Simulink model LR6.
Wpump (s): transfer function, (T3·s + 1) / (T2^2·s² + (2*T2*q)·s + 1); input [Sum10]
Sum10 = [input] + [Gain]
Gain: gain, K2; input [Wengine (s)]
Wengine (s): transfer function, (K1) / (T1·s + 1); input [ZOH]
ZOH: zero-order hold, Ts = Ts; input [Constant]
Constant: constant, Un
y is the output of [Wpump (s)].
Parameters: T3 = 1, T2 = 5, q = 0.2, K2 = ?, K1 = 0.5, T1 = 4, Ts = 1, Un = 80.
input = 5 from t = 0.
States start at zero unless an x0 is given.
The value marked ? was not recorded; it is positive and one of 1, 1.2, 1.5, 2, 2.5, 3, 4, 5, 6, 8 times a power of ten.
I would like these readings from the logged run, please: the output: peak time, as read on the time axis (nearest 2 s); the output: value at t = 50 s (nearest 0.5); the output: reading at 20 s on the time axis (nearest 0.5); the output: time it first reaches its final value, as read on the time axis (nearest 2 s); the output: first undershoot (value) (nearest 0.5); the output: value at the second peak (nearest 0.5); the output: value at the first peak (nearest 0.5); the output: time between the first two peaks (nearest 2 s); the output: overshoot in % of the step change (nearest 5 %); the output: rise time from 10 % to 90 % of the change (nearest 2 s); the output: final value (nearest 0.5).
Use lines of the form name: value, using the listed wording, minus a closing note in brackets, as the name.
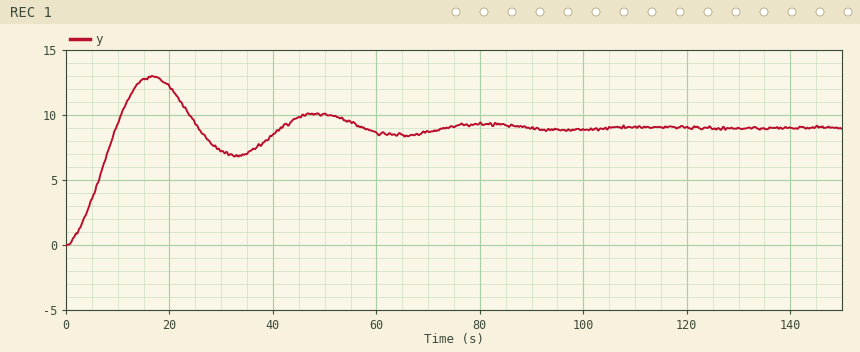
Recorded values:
the output: peak time, as read on the time axis: 16 s
the output: value at t = 50 s: 10.0
the output: reading at 20 s on the time axis: 12.0
the output: time it first reaches its final value, as read on the time axis: 10 s
the output: first undershoot (value): 7.0
the output: value at the second peak: 10.0
the output: value at the first peak: 13.0
the output: time between the first two peaks: 32 s
the output: overshoot in % of the step change: 45 %
the output: rise time from 10 % to 90 % of the change: 6 s
the output: final value: 9.0
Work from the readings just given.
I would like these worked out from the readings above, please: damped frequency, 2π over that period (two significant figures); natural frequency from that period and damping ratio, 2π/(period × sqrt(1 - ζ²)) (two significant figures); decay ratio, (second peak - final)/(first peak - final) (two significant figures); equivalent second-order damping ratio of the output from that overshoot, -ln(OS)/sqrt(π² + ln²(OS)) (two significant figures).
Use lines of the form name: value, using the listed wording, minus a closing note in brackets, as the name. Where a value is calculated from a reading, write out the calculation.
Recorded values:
damped frequency, 2π over that period: 2π / 32 = 0.20 rad/s
natural frequency from that period and damping ratio, 2π/(period × sqrt(1 - ζ²)): 2π / (32 × sqrt(1 - 0.25²)) = 0.20 rad/s
decay ratio, (second peak - final)/(first peak - final): (10 - 9) / (13 - 9) = 0.25
equivalent second-order damping ratio of the output from that overshoot, -ln(OS)/sqrt(π² + ln²(OS)): ln(0.45) = -0.799; 0.799 / sqrt(9.870 + 0.638) = 0.25
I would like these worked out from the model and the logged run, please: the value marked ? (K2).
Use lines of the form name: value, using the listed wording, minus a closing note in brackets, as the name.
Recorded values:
the value marked ?: 0.1
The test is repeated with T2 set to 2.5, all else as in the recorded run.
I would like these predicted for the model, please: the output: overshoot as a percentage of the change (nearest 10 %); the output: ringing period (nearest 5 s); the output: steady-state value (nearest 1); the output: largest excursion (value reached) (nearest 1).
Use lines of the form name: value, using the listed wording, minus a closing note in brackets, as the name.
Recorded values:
the output: overshoot as a percentage of the change: 30 %
the output: ringing period: 15 s
the output: steady-state value: 9
the output: largest excursion (value reached): 12
